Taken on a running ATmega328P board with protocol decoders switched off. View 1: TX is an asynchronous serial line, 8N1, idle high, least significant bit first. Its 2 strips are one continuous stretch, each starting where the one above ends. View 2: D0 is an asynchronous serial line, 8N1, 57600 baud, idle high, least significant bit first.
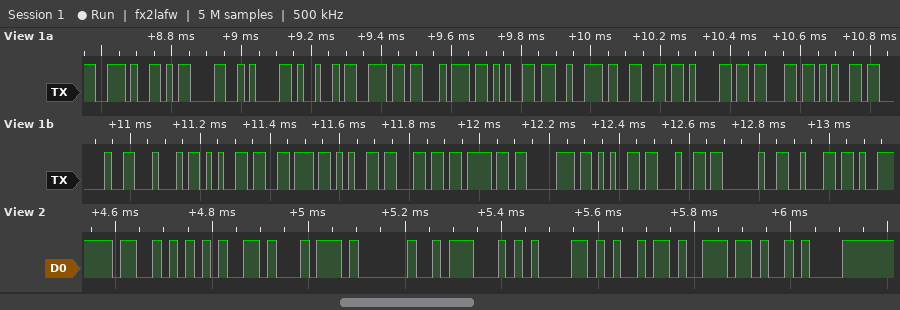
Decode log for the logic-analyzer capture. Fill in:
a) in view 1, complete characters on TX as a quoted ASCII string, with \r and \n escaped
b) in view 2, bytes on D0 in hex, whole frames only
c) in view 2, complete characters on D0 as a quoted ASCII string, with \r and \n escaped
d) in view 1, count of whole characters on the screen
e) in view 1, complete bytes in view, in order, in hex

".\r\nInterface Developed b"
53 65 74 20 47 61 69 6E 0A
"Set Gain\n"
24
2E 0D 0A 49 6E 74 65 72 66 61 63 65 20 44 65 76 65 6C 6F 70 65 64 20 62
